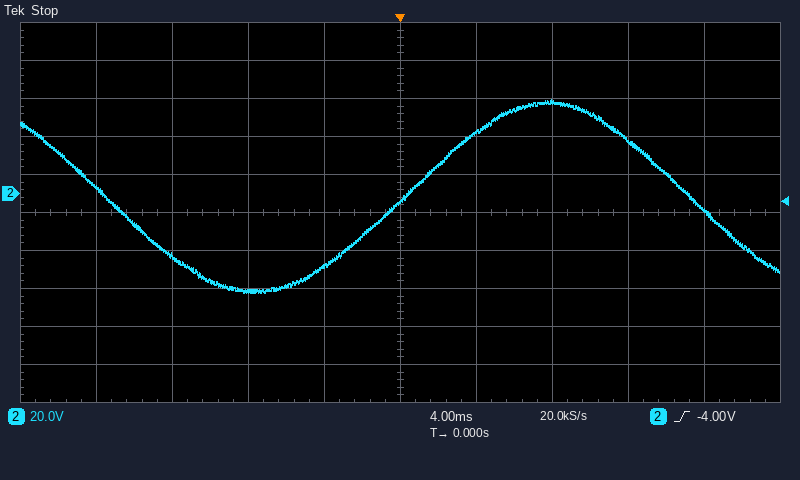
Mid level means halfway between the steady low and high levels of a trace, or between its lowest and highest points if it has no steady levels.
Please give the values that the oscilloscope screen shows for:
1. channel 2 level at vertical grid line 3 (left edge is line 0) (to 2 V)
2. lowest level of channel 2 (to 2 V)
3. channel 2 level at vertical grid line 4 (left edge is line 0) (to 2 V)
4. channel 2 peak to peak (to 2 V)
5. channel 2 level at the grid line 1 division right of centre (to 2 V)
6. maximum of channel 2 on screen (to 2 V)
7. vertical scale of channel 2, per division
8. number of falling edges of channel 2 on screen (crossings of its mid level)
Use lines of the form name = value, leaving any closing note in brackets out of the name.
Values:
channel 2 level at vertical grid line 3 (left edge is line 0) = -52 V
lowest level of channel 2 = -52 V
channel 2 level at vertical grid line 4 (left edge is line 0) = -38 V
channel 2 peak to peak = 102 V
channel 2 level at the grid line 1 division right of centre = 32 V
maximum of channel 2 on screen = 50 V
vertical scale of channel 2, per division = 20 V
number of falling edges of channel 2 on screen = 2
